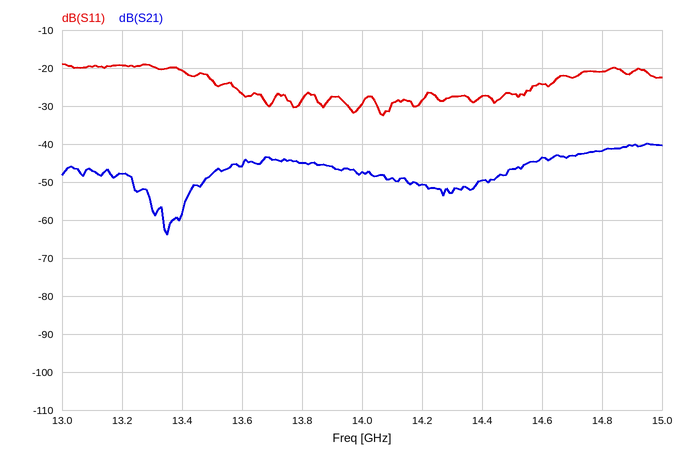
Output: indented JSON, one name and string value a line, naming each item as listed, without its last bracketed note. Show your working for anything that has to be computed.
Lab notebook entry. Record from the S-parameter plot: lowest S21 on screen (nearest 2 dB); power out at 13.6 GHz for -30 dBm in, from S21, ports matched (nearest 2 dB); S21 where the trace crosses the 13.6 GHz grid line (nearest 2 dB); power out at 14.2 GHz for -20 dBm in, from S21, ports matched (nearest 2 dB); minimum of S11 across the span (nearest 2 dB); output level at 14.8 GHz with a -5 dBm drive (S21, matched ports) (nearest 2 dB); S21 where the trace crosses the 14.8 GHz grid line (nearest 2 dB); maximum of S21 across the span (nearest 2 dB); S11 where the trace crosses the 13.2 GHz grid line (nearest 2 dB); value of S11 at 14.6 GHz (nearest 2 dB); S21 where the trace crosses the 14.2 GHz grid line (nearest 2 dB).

{
  "lowest S21 on screen": "-64 dB",
  "power out at 13.6 GHz for -30 dBm in, from S21, ports matched": "-30 dBm + (-46 dB) = -76 dBm",
  "S21 where the trace crosses the 13.6 GHz grid line": "-46 dB",
  "power out at 14.2 GHz for -20 dBm in, from S21, ports matched": "-20 dBm + (-50 dB) = -70 dBm",
  "minimum of S11 across the span": "-32 dB",
  "output level at 14.8 GHz with a -5 dBm drive (S21, matched ports)": "-5 dBm + (-42 dB) = -46 dBm",
  "S21 where the trace crosses the 14.8 GHz grid line": "-42 dB",
  "maximum of S21 across the span": "-40 dB",
  "S11 where the trace crosses the 13.2 GHz grid line": "-20 dB",
  "value of S11 at 14.6 GHz": "-24 dB",
  "S21 where the trace crosses the 14.2 GHz grid line": "-50 dB"
}
